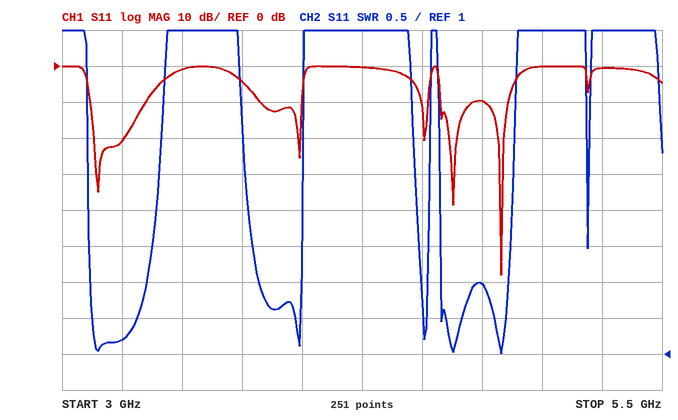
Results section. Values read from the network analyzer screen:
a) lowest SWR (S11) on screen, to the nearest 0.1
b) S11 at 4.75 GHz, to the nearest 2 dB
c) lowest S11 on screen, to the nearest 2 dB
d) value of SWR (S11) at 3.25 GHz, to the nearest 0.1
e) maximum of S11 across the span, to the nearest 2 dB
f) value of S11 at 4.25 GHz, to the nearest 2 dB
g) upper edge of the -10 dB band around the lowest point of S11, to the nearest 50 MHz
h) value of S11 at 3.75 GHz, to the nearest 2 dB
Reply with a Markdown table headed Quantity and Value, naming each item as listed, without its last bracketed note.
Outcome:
| Quantity | Value |
|---|---|
| lowest SWR (S11) on screen, to the nearest 0.1 | 1.0 |
| S11 at 4.75 GHz, to the nearest 2 dB | -10 dB |
| lowest S11 on screen, to the nearest 2 dB | -58 dB |
| value of SWR (S11) at 3.25 GHz, to the nearest 0.1 | 1.2 |
| maximum of S11 across the span, to the nearest 2 dB | 0 dB |
| value of S11 at 4.25 GHz, to the nearest 2 dB | 0 dB |
| upper edge of the -10 dB band around the lowest point of S11, to the nearest 50 MHz | 4.85 GHz |
| value of S11 at 3.75 GHz, to the nearest 2 dB | -4 dB |
